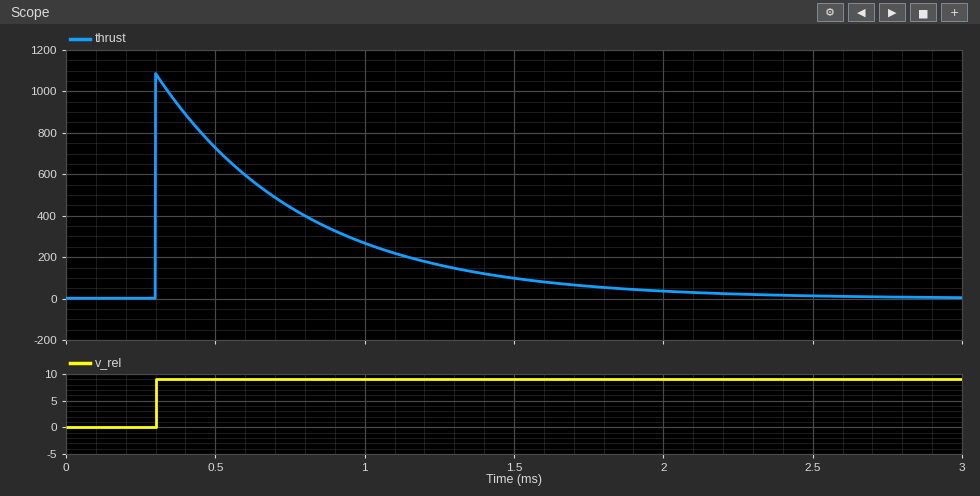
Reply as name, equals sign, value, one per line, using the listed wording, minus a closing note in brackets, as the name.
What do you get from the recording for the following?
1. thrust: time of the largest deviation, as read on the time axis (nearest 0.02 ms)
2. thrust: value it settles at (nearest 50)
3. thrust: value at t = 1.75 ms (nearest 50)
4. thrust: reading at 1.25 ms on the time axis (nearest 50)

thrust: time of the largest deviation, as read on the time axis = 0.30 ms
thrust: value it settles at = 0
thrust: value at t = 1.75 ms = 50
thrust: reading at 1.25 ms on the time axis = 150
